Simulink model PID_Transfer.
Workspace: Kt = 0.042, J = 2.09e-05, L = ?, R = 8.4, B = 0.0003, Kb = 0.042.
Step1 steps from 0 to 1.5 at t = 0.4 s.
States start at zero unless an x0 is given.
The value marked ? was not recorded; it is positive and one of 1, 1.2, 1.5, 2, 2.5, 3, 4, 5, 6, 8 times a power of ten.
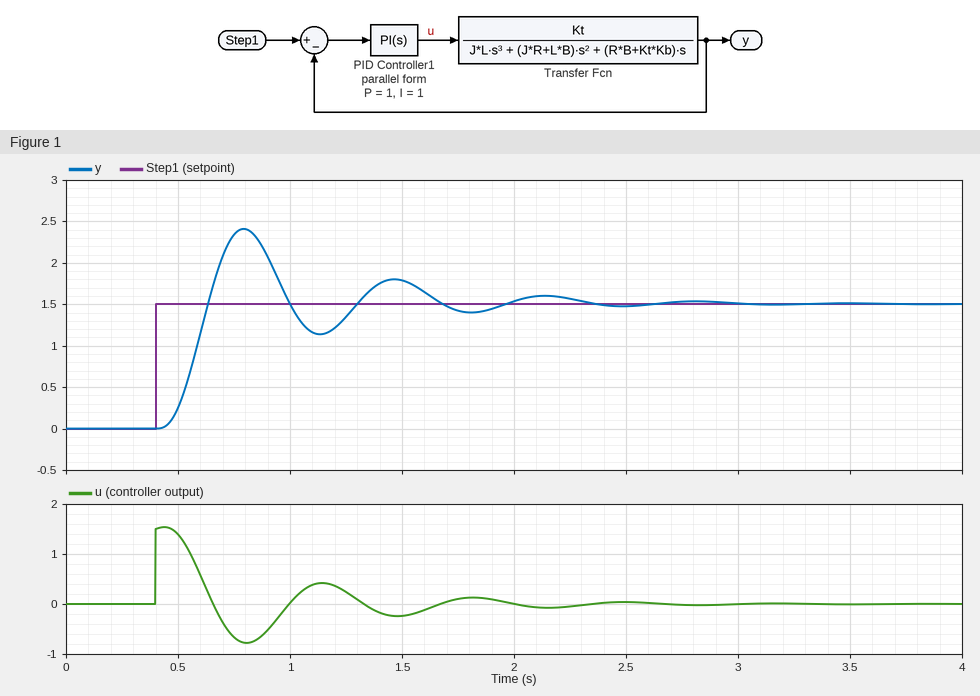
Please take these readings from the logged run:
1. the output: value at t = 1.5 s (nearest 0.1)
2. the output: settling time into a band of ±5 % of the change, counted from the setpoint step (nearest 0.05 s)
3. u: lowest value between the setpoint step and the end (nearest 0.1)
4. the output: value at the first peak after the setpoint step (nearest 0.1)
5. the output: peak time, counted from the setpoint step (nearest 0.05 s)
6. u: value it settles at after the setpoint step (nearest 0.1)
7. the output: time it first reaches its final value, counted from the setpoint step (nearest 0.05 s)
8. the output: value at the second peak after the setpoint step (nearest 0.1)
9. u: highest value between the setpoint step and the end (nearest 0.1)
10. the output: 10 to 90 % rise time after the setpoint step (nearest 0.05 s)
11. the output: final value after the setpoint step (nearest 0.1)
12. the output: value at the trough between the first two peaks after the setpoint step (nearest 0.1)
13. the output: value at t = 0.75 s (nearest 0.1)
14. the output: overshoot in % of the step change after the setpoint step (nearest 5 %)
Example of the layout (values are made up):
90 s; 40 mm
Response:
1.8; 1.85 s; -0.8; 2.4; 0.40 s; 0.0; 0.25 s; 1.8; 1.5; 0.15 s; 1.5; 1.1; 2.3; 60 %
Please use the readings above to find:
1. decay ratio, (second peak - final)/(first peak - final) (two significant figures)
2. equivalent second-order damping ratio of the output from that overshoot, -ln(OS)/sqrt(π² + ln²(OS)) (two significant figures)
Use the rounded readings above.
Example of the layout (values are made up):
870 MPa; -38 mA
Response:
0.33; 0.16
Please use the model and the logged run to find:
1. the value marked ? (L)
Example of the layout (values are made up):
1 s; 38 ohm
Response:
1.2
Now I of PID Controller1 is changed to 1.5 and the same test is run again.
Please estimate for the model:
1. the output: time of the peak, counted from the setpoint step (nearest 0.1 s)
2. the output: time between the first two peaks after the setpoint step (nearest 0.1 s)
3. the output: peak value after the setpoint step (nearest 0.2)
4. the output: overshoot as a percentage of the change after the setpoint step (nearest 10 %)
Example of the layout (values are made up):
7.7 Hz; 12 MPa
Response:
0.4 s; 0.7 s; 2.6; 70 %
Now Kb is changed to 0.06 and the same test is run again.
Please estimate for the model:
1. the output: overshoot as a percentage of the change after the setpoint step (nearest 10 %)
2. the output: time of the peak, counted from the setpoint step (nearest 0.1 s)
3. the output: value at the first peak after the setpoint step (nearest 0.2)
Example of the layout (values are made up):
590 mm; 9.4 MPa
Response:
50 %; 0.4 s; 2.2
